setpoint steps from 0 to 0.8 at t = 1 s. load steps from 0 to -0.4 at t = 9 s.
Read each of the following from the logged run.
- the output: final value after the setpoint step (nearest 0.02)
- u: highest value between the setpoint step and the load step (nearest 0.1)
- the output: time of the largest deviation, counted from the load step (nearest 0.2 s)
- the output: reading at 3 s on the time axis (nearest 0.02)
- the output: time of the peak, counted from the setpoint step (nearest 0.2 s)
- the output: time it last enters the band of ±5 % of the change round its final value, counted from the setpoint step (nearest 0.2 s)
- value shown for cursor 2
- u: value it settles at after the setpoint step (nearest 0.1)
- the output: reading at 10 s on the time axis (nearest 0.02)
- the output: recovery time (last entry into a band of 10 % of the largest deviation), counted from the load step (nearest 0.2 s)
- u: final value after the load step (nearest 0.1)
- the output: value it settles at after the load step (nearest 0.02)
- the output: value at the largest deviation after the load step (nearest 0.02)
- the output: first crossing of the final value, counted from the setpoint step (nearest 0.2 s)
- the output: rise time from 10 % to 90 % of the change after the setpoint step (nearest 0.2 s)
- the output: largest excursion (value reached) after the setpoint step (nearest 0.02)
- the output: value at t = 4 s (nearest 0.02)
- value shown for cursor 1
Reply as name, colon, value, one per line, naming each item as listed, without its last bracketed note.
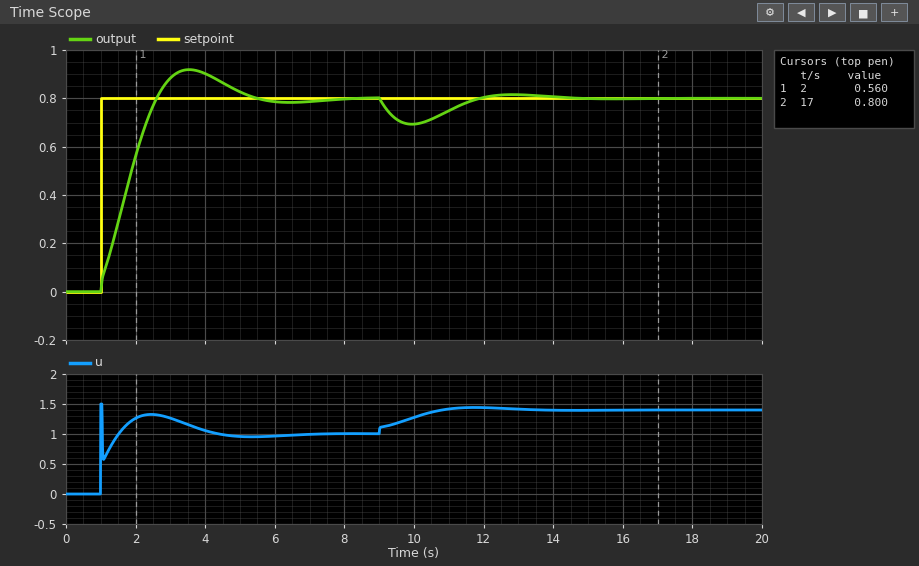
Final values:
the output: final value after the setpoint step: 0.80
u: highest value between the setpoint step and the load step: 1.5
the output: time of the largest deviation, counted from the load step: 1.0 s
the output: reading at 3 s on the time axis: 0.88
the output: time of the peak, counted from the setpoint step: 2.6 s
the output: time it last enters the band of ±5 % of the change round its final value, counted from the setpoint step: 3.8 s
value shown for cursor 2: 0.800
u: value it settles at after the setpoint step: 1.0
the output: reading at 10 s on the time axis: 0.70
the output: recovery time (last entry into a band of 10 % of the largest deviation), counted from the load step: 4.6 s
u: final value after the load step: 1.4
the output: value it settles at after the load step: 0.80
the output: value at the largest deviation after the load step: 0.70
the output: first crossing of the final value, counted from the setpoint step: 1.6 s
the output: rise time from 10 % to 90 % of the change after the setpoint step: 1.2 s
the output: largest excursion (value reached) after the setpoint step: 0.92
the output: value at t = 4 s: 0.90
value shown for cursor 1: 0.560
